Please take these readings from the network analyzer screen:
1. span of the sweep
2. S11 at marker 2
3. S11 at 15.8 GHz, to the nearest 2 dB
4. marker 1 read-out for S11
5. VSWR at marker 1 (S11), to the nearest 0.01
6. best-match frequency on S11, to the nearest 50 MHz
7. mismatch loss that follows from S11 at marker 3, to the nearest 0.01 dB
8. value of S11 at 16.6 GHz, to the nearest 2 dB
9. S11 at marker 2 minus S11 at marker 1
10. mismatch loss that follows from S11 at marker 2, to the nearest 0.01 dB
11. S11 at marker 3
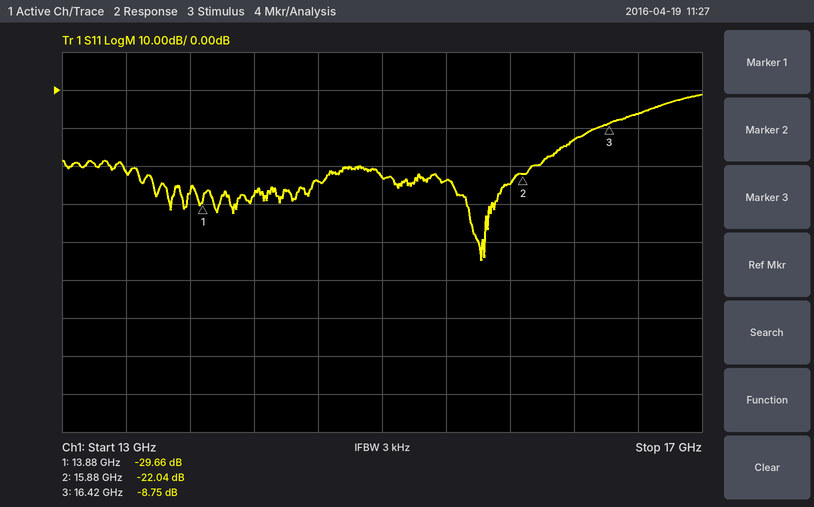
4 GHz
-22.04 dB
-24 dB
-29.66 dB
1.07
15.60 GHz
0.62 dB
-6 dB
7.62 dB
0.03 dB
-8.75 dB
